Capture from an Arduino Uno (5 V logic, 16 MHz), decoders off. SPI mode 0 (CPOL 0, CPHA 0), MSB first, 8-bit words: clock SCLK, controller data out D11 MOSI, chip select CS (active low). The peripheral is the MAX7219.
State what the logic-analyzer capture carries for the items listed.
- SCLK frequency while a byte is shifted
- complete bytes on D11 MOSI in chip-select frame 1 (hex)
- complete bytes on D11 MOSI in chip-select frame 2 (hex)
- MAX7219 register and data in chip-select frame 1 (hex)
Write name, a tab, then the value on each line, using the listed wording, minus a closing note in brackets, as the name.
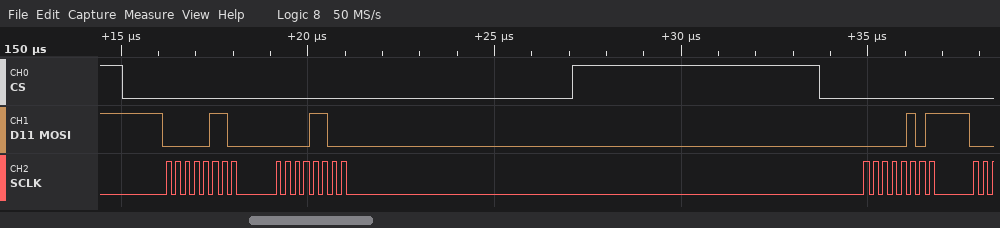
SCLK frequency while a byte is shifted	4 MHz
complete bytes on D11 MOSI in chip-select frame 1	06 0C
complete bytes on D11 MOSI in chip-select frame 2	05
MAX7219 register and data in chip-select frame 1	register 0x6, data 0x0C
